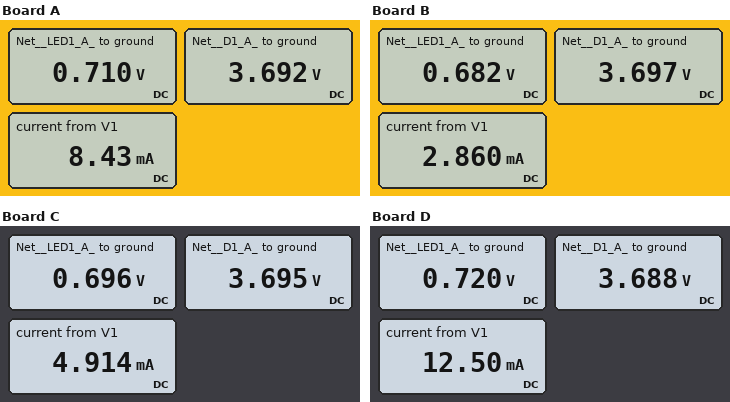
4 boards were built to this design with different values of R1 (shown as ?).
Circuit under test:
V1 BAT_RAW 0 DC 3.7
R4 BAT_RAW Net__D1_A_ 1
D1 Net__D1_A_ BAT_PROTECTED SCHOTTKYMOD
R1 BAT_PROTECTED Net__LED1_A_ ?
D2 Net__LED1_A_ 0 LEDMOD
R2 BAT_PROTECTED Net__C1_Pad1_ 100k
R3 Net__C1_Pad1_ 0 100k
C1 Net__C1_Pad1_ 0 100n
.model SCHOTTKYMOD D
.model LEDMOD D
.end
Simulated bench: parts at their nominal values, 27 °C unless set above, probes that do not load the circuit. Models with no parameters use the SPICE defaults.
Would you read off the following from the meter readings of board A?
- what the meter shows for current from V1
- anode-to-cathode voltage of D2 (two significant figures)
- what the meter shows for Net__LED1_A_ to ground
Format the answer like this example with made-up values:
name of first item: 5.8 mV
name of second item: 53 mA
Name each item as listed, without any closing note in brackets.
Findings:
what the meter shows for current from V1: 8.43 mA
anode-to-cathode voltage of D2: 710 mV
what the meter shows for Net__LED1_A_ to ground: 0.710 V
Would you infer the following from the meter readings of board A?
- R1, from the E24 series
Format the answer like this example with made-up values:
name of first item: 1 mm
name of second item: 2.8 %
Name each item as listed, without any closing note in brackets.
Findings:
R1, from the E24 series: 270 Ω
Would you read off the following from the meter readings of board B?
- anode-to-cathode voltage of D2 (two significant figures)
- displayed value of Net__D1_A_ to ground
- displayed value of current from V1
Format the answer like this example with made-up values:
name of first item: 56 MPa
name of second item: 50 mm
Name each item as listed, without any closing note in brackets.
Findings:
anode-to-cathode voltage of D2: 680 mV
displayed value of Net__D1_A_ to ground: 3.697 V
displayed value of current from V1: 2.860 mA
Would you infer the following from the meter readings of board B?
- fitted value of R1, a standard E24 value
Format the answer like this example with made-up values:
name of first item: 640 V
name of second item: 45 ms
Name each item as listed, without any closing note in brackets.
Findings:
fitted value of R1, a standard E24 value: 820 Ω
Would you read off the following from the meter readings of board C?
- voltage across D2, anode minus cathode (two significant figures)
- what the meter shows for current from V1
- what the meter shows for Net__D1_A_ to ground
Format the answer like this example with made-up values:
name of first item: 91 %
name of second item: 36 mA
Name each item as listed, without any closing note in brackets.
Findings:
voltage across D2, anode minus cathode: 700 mV
what the meter shows for current from V1: 4.914 mA
what the meter shows for Net__D1_A_ to ground: 3.695 V
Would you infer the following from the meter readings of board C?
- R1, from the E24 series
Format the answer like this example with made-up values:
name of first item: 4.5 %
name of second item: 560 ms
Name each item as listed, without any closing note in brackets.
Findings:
R1, from the E24 series: 470 Ω
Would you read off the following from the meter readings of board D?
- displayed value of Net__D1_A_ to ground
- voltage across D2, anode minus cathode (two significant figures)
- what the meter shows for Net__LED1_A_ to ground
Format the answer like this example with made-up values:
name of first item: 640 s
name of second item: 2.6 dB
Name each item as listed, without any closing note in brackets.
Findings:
displayed value of Net__D1_A_ to ground: 3.688 V
voltage across D2, anode minus cathode: 720 mV
what the meter shows for Net__LED1_A_ to ground: 0.720 V
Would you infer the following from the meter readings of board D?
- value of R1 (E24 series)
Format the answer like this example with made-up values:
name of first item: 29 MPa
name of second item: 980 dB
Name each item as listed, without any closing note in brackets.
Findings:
value of R1: 180 Ω
